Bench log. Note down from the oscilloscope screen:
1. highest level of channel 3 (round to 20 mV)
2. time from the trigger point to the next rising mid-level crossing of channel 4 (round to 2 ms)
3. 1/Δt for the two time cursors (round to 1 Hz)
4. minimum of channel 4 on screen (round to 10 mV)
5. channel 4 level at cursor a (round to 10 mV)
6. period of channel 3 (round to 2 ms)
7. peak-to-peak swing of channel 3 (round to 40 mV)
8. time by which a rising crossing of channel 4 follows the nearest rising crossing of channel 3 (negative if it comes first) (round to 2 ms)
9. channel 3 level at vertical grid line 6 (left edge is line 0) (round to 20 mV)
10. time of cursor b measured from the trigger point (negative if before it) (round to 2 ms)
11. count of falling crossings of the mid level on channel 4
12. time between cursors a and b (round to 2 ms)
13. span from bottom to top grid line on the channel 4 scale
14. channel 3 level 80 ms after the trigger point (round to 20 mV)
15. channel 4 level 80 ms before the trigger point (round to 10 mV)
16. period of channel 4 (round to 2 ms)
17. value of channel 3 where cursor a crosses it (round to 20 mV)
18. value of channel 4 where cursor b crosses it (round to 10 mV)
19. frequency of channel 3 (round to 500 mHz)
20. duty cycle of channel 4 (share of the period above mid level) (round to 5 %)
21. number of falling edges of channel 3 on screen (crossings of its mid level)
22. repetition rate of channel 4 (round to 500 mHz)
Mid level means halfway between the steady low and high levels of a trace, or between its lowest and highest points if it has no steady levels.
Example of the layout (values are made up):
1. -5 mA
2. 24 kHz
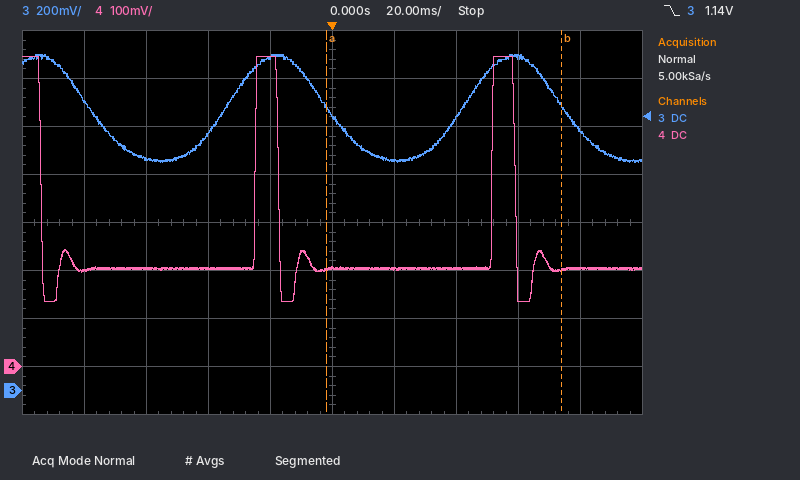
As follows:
1. 1.40 V
2. 52 ms
3. 13 Hz
4. 140 mV
5. 200 mV
6. 76 ms
7. 440 mV
8. +10 ms
9. 960 mV
10. +74 ms
11. 3
12. 76 ms
13. 800 mV
14. 1.08 V
15. 200 mV
16. 76 ms
17. 1.18 V
18. 200 mV
19. 13.0 Hz
20. 10 %
21. 3
22. 13.0 Hz
